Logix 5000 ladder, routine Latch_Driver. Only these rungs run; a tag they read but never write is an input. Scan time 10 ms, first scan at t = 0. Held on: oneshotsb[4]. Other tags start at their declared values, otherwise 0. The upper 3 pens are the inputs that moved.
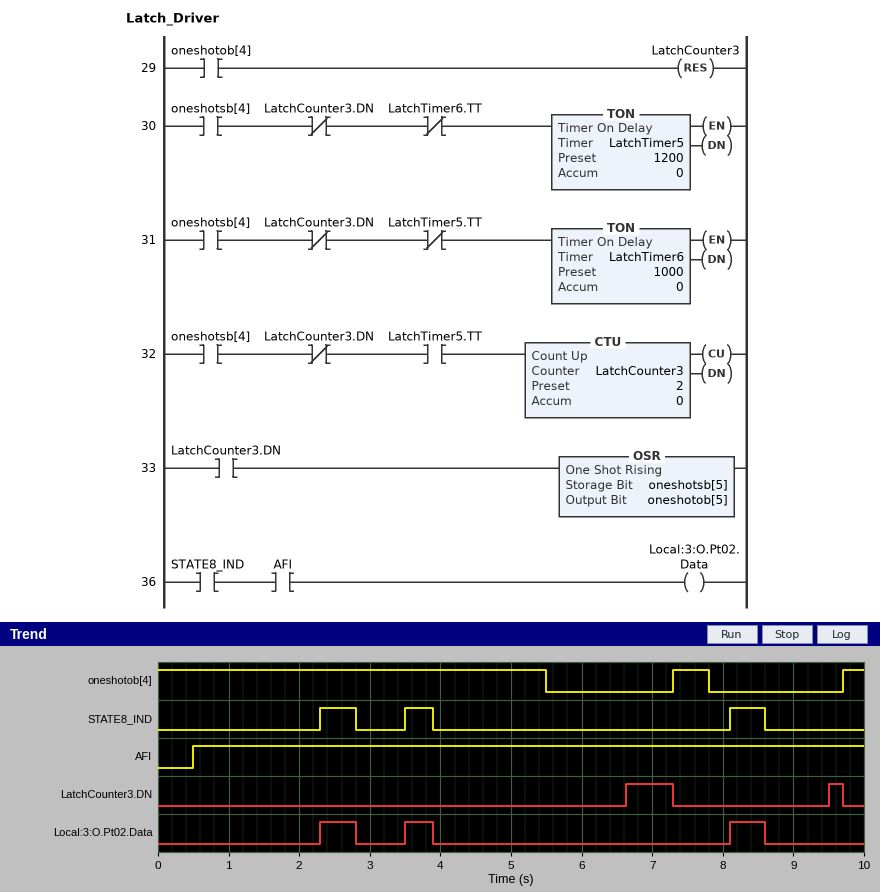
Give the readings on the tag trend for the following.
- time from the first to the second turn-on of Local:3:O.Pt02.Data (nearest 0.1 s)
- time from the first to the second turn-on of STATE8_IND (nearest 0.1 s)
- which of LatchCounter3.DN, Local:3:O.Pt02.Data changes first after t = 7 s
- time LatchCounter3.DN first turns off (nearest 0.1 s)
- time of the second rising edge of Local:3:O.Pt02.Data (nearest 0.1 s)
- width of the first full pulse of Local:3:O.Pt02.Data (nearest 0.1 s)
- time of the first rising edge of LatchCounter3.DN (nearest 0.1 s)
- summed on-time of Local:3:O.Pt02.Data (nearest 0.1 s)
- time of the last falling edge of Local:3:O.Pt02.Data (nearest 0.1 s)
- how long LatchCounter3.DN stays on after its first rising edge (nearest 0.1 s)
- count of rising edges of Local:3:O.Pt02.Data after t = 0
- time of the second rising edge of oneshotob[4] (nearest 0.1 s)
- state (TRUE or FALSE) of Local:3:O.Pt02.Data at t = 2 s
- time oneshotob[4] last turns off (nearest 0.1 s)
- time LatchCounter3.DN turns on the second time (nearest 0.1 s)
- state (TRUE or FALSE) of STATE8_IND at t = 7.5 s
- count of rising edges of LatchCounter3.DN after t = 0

1.2 s
1.2 s
LatchCounter3.DN
7.3 s
3.5 s
0.5 s
6.6 s
1.4 s
8.6 s
0.7 s
3
9.7 s
FALSE
7.8 s
9.5 s
FALSE
2
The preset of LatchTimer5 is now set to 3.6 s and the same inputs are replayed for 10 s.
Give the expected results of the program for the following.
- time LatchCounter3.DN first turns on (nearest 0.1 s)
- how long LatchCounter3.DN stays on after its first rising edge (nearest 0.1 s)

9.2 s
0.5 s
